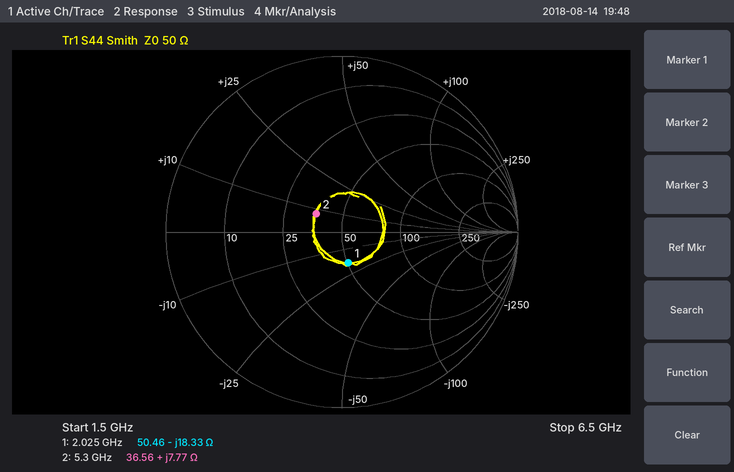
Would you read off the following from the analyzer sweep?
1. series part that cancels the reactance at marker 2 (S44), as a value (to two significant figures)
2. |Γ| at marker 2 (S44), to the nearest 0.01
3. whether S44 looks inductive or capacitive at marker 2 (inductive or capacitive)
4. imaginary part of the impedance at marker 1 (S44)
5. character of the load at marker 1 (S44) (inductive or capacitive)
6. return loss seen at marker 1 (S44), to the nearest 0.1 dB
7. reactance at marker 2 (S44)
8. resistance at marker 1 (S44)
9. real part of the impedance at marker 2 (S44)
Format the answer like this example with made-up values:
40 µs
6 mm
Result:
3.9 pF
0.18
inductive
-18.33 Ω
capacitive
14.9 dB
+7.77 Ω
50.46 Ω
36.56 Ω
